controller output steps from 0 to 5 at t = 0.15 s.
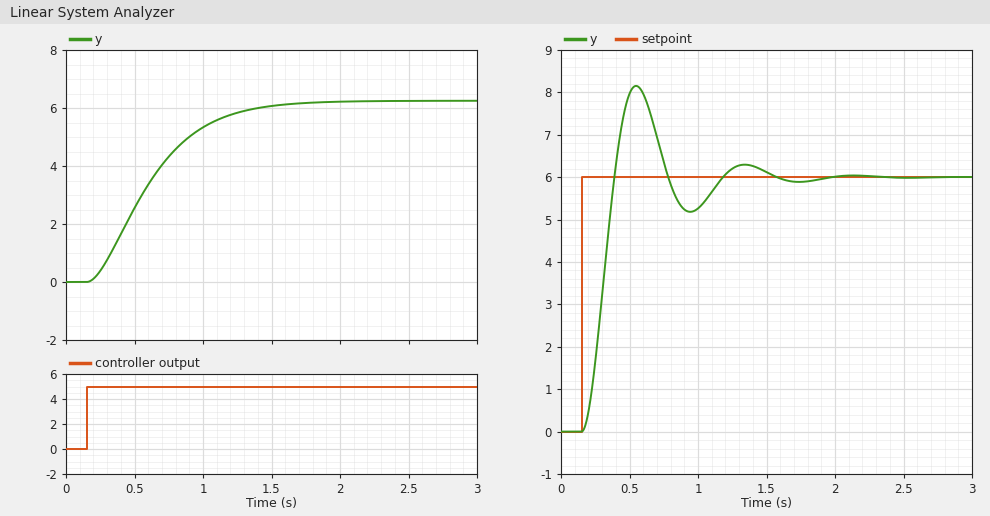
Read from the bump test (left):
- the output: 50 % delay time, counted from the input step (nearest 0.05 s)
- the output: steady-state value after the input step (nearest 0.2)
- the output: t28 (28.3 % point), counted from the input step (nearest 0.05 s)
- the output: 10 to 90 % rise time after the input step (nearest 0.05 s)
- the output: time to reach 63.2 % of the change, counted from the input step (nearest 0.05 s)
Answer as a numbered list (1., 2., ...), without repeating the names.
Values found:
1. 0.40 s
2. 6.2
3. 0.25 s
4. 0.85 s
5. 0.55 s
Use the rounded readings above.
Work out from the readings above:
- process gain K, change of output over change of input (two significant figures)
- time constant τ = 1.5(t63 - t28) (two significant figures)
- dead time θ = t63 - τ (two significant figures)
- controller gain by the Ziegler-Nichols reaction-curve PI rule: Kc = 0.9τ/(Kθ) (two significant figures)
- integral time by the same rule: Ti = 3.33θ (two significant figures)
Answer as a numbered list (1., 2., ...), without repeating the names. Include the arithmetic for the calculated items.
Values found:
1. (6.2 - 0) / 5 = 1.2
2. 1.5 × (0.55 - 0.25) = 0.45 s
3. 0.55 - 0.45 = 0.10 s
4. 0.9 × 0.45 / (1.2 × 0.1) = 3.4
5. 3.33 × 0.1 = 0.33 s
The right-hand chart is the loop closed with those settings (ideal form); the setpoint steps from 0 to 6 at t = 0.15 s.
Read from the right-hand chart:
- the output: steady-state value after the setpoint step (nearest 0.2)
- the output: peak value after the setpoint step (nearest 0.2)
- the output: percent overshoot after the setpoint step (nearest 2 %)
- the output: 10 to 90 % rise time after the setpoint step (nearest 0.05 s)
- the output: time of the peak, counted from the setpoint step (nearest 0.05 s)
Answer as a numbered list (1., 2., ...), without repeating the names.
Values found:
1. 6.0
2. 8.2
3. 36 %
4. 0.15 s
5. 0.40 s
